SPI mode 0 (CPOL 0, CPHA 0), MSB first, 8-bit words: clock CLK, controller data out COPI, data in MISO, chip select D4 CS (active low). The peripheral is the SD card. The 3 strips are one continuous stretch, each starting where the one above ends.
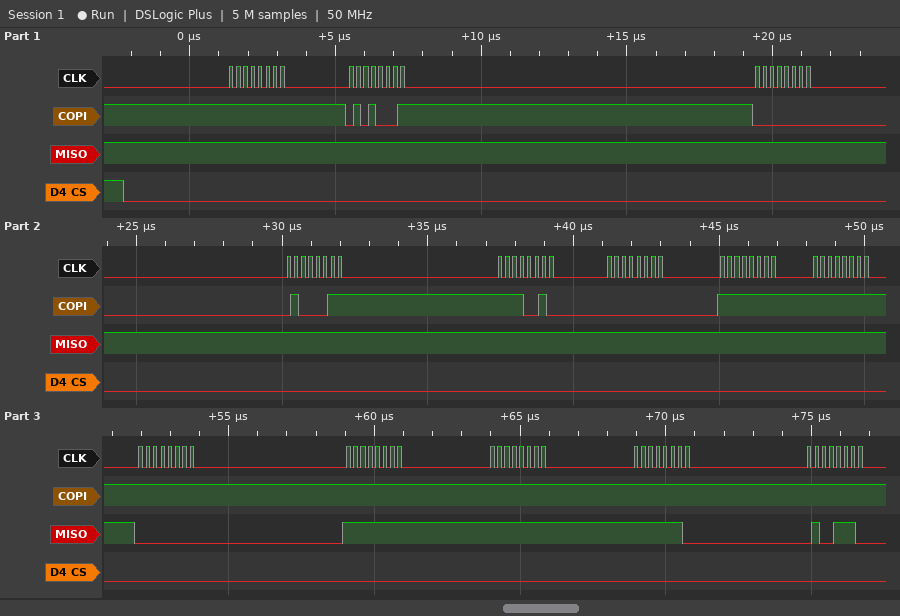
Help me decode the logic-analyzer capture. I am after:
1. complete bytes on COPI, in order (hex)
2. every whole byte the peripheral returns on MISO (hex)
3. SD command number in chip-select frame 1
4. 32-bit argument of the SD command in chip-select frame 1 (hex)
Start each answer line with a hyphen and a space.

- FF 51 00 43 F2 00 FF FF FF FF FF FF FF
- FF FF FF FF FF FF FF FF 00 FF FF FE 4E
- CMD17
- 0x0043F200
